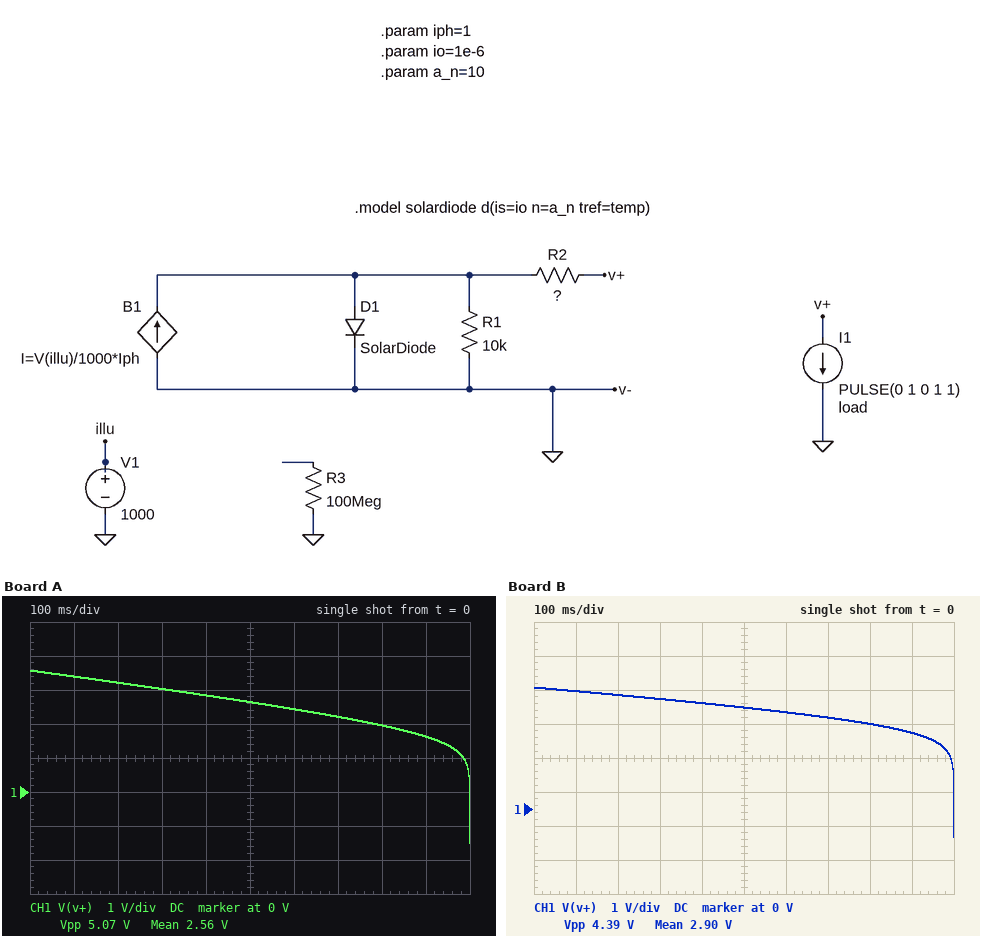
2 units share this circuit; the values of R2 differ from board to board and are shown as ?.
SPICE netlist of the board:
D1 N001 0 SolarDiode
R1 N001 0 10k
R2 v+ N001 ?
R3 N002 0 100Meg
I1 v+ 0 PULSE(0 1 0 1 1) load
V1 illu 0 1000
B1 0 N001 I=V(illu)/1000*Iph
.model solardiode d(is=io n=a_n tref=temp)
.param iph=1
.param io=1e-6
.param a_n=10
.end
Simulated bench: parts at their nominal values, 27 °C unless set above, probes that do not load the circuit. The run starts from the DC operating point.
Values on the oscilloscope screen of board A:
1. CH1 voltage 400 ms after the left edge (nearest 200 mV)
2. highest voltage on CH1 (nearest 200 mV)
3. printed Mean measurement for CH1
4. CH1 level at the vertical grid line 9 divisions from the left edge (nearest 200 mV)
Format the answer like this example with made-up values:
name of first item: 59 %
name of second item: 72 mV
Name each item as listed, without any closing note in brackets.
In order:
CH1 voltage 400 ms after the left edge: 2.8 V
highest voltage on CH1: 3.6 V
printed Mean measurement for CH1: 2.56 V
CH1 level at the vertical grid line 9 divisions from the left edge: 1.6 V
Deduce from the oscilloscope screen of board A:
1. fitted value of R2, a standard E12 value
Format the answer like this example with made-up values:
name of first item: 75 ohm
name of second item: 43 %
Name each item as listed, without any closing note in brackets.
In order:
fitted value of R2, a standard E12 value: 1.5 Ω
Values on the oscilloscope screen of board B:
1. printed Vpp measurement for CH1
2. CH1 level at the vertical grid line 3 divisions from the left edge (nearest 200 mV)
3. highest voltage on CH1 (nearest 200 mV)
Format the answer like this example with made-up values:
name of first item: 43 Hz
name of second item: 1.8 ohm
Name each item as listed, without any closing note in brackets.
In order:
printed Vpp measurement for CH1: 4.39 V
CH1 level at the vertical grid line 3 divisions from the left edge: 3.2 V
highest voltage on CH1: 3.6 V
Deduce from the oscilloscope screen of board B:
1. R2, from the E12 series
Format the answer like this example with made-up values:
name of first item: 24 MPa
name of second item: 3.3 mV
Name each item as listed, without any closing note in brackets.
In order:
R2, from the E12 series: 0.82 Ω
